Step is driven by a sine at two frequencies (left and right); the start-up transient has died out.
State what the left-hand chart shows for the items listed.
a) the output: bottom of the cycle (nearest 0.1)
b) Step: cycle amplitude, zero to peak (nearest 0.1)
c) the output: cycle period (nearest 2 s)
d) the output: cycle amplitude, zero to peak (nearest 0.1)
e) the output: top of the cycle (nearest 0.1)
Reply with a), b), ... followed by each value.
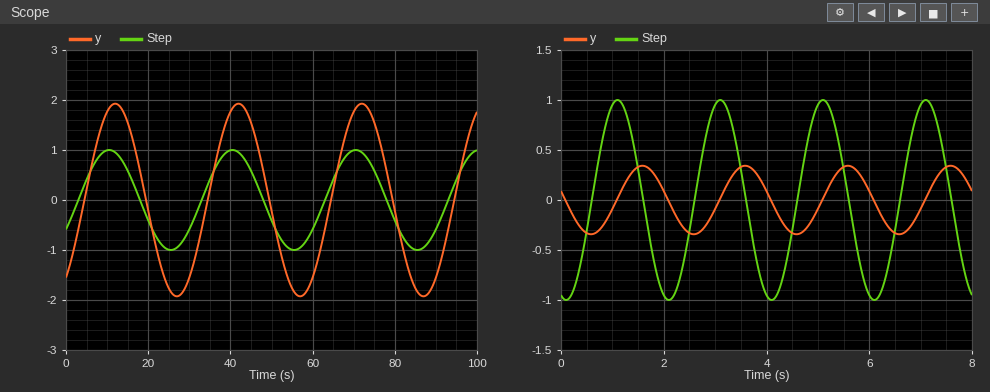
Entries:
a) -1.9
b) 1.0
c) 30 s
d) 1.9
e) 1.9
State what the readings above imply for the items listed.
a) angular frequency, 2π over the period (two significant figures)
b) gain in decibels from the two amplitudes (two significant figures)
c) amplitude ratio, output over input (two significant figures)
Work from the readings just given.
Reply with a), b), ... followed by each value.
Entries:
a) 0.21 rad/s
b) 5.6 dB
c) 1.9
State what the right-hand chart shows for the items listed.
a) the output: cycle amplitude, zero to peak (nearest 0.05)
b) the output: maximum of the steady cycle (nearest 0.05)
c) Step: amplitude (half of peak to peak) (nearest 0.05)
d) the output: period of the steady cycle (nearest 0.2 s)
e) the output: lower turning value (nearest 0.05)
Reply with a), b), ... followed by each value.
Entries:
a) 0.35
b) 0.35
c) 1.00
d) 2.0 s
e) -0.35
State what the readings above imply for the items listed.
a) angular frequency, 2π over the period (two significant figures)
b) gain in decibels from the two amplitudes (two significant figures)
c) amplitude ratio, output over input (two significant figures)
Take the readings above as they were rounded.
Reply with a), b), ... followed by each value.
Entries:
a) 3.1 rad/s
b) -9.1 dB
c) 0.35
